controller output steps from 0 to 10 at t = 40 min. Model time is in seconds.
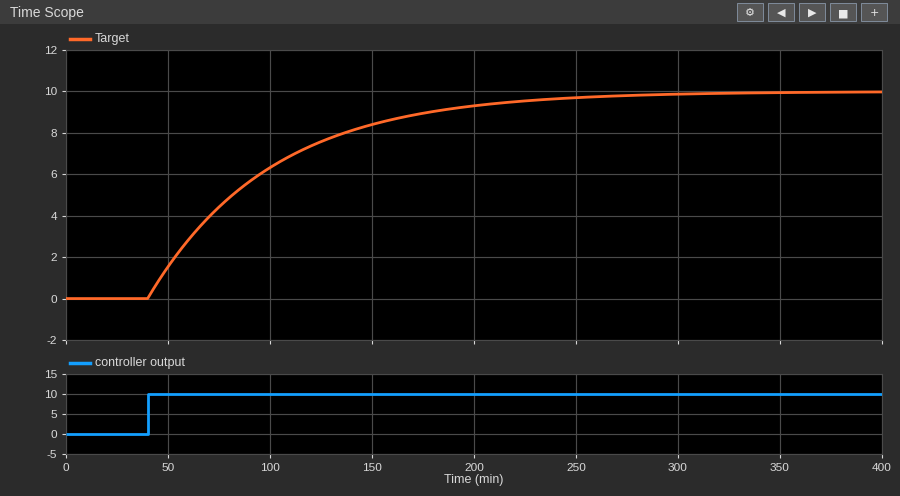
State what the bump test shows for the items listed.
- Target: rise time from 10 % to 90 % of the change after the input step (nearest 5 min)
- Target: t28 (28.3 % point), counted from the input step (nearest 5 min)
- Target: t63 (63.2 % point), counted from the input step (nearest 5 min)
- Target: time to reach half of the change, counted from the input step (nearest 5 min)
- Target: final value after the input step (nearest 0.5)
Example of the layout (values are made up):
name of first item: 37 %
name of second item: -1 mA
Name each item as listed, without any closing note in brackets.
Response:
Target: rise time from 10 % to 90 % of the change after the input step: 130 min
Target: t28 (28.3 % point), counted from the input step: 20 min
Target: t63 (63.2 % point), counted from the input step: 60 min
Target: time to reach half of the change, counted from the input step: 40 min
Target: final value after the input step: 10.0
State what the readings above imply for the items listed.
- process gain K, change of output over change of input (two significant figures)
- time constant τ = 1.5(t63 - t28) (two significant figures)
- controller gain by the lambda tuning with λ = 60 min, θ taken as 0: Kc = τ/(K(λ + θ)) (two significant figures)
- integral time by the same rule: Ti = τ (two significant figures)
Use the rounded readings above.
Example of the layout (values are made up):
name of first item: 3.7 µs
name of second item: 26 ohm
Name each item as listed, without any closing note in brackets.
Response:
process gain K, change of output over change of input: 1.0
time constant τ = 1.5(t63 - t28): 60 min
controller gain by the lambda tuning with λ = 60 min, θ taken as 0: Kc = τ/(K(λ + θ)): 1.0
integral time by the same rule: Ti = τ: 60 min
